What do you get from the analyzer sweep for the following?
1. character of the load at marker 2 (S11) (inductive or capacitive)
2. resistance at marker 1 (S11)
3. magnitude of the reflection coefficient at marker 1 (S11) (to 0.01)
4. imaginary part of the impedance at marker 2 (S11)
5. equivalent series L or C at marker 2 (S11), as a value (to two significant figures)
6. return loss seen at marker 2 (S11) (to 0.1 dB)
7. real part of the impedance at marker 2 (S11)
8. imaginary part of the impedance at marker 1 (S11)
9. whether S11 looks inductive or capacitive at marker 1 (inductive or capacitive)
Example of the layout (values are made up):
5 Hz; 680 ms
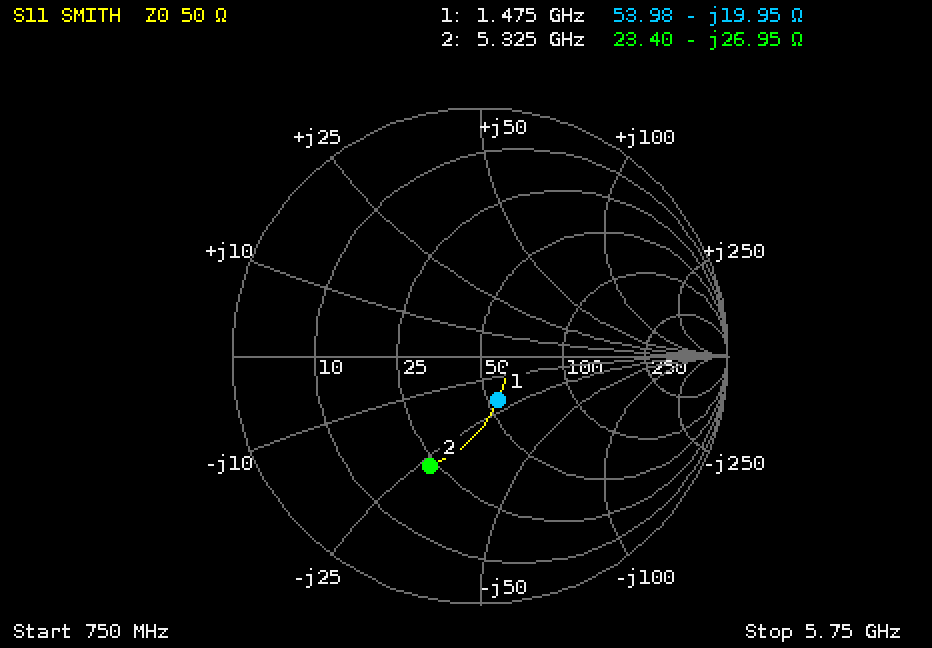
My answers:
capacitive; 53.98 Ω; 0.19; -26.95 Ω; 1.1 pF; 6.3 dB; 23.40 Ω; -19.95 Ω; capacitive
